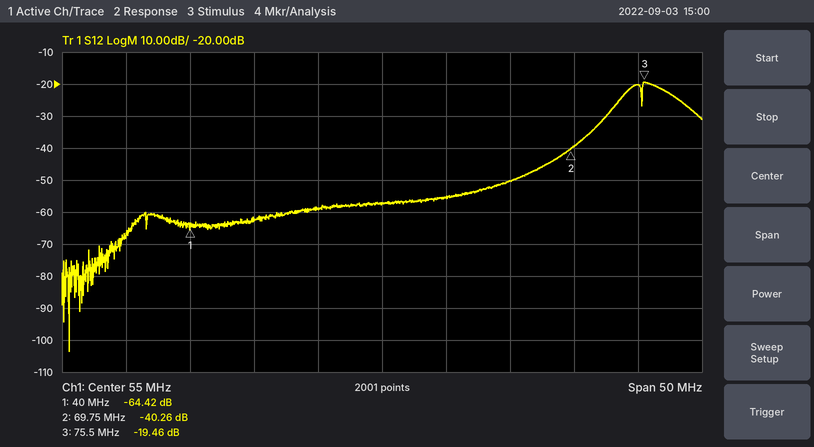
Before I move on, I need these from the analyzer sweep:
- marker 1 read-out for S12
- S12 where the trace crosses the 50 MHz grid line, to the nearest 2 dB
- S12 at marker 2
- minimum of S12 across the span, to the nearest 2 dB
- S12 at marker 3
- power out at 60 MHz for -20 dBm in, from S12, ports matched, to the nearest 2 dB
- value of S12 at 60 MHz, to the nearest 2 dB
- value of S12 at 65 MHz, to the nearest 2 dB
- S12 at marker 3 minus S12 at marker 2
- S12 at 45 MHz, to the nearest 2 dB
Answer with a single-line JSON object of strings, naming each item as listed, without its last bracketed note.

{"marker 1 read-out for S12": "-64.42 dB", "S12 where the trace crosses the 50 MHz grid line, to the nearest 2 dB": "-58 dB", "S12 at marker 2": "-40.26 dB", "minimum of S12 across the span, to the nearest 2 dB": "-104 dB", "S12 at marker 3": "-19.46 dB", "power out at 60 MHz for -20 dBm in, from S12, ports matched, to the nearest 2 dB": "-76 dBm", "value of S12 at 60 MHz, to the nearest 2 dB": "-56 dB", "value of S12 at 65 MHz, to the nearest 2 dB": "-50 dB", "S12 at marker 3 minus S12 at marker 2": "20.80 dB", "S12 at 45 MHz, to the nearest 2 dB": "-62 dB"}
